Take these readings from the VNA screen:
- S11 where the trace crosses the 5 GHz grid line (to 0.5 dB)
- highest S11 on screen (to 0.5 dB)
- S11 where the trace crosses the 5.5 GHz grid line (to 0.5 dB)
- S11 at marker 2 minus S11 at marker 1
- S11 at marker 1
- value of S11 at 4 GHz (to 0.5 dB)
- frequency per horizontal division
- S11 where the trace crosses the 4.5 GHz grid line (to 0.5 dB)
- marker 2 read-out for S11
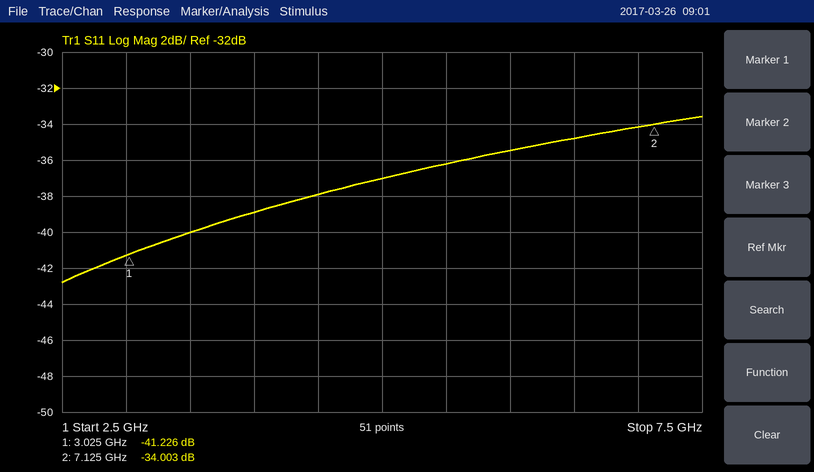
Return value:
-37.0 dB
-33.5 dB
-36.0 dB
7.223 dB
-41.226 dB
-39.0 dB
500 MHz
-38.0 dB
-34.003 dB
